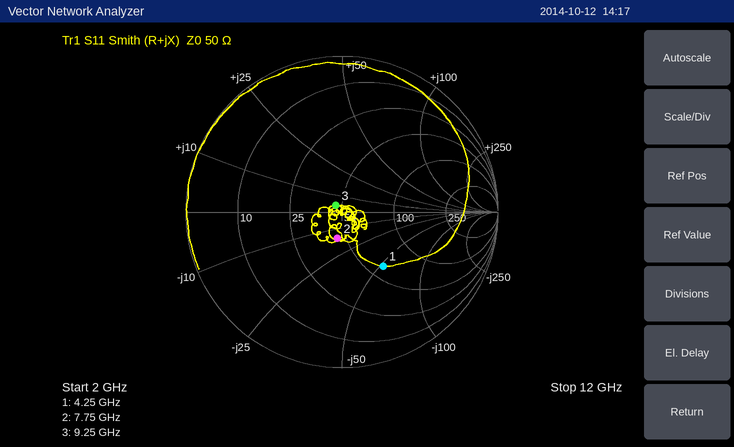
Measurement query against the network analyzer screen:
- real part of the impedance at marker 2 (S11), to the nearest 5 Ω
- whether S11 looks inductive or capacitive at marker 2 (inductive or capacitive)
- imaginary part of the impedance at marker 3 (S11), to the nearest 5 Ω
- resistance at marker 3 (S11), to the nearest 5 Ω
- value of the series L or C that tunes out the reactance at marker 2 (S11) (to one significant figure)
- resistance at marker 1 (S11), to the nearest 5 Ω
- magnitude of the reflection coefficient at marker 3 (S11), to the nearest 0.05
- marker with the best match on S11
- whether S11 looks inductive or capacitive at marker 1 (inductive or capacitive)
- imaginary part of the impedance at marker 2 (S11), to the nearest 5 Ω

45 Ω
capacitive
+5 Ω
45 Ω
300 pH
60 Ω
0.05
marker 3
capacitive
-15 Ω
